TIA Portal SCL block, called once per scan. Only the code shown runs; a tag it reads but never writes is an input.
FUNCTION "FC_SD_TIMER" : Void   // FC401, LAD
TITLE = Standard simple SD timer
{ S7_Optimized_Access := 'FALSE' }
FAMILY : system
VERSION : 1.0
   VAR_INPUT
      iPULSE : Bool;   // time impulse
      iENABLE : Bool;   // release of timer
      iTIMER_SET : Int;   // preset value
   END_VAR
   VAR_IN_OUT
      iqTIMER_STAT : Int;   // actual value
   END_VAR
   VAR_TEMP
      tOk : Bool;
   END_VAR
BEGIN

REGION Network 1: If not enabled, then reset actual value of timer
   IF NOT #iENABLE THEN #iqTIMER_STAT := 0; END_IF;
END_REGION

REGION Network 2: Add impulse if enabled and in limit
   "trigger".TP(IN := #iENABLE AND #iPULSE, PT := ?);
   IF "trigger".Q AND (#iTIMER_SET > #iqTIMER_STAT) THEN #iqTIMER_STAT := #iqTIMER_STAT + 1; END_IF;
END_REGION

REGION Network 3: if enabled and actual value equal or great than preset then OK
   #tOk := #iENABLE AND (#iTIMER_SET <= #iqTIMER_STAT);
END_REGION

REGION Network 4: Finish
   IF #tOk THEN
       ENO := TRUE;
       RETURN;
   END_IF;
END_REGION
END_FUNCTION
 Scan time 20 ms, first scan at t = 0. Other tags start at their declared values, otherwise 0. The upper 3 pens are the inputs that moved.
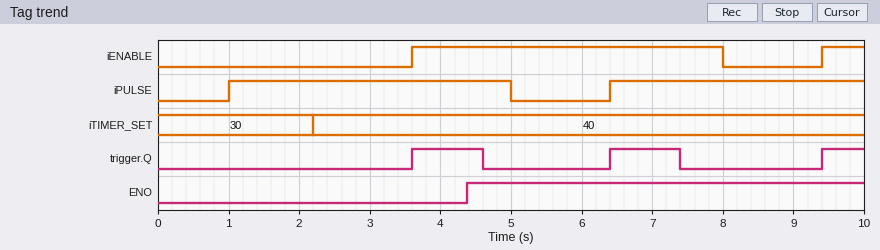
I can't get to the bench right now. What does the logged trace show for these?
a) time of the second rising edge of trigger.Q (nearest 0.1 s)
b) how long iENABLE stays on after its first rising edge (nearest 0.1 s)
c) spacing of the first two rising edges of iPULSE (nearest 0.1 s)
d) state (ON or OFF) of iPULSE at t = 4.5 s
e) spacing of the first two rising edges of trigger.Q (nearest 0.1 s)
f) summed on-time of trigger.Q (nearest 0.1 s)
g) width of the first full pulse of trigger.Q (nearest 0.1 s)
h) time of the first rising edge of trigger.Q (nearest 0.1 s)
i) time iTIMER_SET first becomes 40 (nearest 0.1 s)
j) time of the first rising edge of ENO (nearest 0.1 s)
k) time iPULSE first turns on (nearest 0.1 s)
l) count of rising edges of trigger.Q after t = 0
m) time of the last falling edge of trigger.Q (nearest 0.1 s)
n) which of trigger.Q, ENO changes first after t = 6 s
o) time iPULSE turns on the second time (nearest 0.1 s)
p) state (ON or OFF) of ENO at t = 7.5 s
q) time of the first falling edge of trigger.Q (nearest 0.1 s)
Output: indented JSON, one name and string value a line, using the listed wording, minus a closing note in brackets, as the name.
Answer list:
{
  "time of the second rising edge of trigger.Q": "6.4 s",
  "how long iENABLE stays on after its first rising edge": "4.4 s",
  "spacing of the first two rising edges of iPULSE": "5.4 s",
  "state (ON or OFF) of iPULSE at t = 4.5 s": "ON",
  "spacing of the first two rising edges of trigger.Q": "2.8 s",
  "summed on-time of trigger.Q": "2.6 s",
  "width of the first full pulse of trigger.Q": "1.0 s",
  "time of the first rising edge of trigger.Q": "3.6 s",
  "time iTIMER_SET first becomes 40": "2.2 s",
  "time of the first rising edge of ENO": "4.4 s",
  "time iPULSE first turns on": "1.0 s",
  "count of rising edges of trigger.Q after t = 0": "3",
  "time of the last falling edge of trigger.Q": "7.4 s",
  "which of trigger.Q, ENO changes first after t = 6 s": "trigger.Q",
  "time iPULSE turns on the second time": "6.4 s",
  "state (ON or OFF) of ENO at t = 7.5 s": "ON",
  "time of the first falling edge of trigger.Q": "4.6 s"
}
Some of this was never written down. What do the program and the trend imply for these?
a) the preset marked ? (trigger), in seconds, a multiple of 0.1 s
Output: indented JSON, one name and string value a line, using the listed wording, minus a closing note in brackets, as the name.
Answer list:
{
  "the preset marked ? (trigger), in seconds, a multiple of 0.1 s": "1.0 s"
}
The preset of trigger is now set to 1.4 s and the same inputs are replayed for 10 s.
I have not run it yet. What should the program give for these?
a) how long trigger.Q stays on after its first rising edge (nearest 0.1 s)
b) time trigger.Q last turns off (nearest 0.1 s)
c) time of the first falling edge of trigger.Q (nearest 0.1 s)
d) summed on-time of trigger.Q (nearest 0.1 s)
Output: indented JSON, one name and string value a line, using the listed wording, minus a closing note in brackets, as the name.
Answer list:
{
  "how long trigger.Q stays on after its first rising edge": "1.4 s",
  "time trigger.Q last turns off": "7.8 s",
  "time of the first falling edge of trigger.Q": "5.0 s",
  "summed on-time of trigger.Q": "3.4 s"
}
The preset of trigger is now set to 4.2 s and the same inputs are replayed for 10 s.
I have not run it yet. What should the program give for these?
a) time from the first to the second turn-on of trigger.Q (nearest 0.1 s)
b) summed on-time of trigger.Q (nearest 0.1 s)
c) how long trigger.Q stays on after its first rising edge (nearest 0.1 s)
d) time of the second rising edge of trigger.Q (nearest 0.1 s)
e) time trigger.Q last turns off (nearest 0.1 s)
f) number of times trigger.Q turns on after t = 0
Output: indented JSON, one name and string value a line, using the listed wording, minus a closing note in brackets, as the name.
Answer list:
{
  "time from the first to the second turn-on of trigger.Q": "5.8 s",
  "summed on-time of trigger.Q": "4.8 s",
  "how long trigger.Q stays on after its first rising edge": "4.2 s",
  "time of the second rising edge of trigger.Q": "9.4 s",
  "time trigger.Q last turns off": "7.8 s",
  "number of times trigger.Q turns on after t = 0": "2"
}
